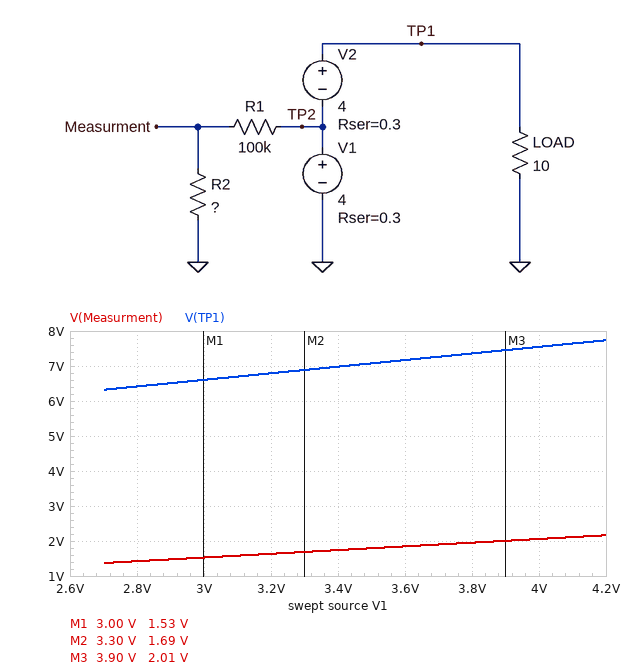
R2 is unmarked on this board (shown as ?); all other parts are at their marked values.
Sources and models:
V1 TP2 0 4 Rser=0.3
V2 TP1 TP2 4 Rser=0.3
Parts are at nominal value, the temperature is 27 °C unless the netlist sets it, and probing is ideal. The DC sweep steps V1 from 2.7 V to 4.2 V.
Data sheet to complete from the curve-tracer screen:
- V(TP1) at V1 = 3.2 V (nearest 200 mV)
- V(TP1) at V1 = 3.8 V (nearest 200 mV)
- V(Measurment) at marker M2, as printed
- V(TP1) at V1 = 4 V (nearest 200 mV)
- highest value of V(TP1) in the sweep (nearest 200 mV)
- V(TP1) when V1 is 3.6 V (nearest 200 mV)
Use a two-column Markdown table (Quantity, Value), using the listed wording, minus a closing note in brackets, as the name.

| Quantity | Value |
|---|---|
| V(TP1) at V1 = 3.2 V | 6.8 V |
| V(TP1) at V1 = 3.8 V | 7.4 V |
| V(Measurment) at marker M2, as printed | 1.69 V |
| V(TP1) at V1 = 4 V | 7.6 V |
| highest value of V(TP1) in the sweep | 7.8 V |
| V(TP1) when V1 is 3.6 V | 7.2 V |
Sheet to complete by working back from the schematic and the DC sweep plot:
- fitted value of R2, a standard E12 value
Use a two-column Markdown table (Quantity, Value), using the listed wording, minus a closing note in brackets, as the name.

| Quantity | Value |
|---|---|
| fitted value of R2, a standard E12 value | 120 kΩ |
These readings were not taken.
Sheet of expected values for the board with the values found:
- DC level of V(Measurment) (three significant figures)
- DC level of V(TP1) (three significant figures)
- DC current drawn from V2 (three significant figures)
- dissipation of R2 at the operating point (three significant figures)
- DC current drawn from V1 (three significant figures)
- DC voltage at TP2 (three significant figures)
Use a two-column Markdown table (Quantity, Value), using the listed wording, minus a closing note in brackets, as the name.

| Quantity | Value |
|---|---|
| DC level of V(Measurment) | 2.06 V |
| DC level of V(TP1) | 7.55 V |
| DC current drawn from V2 | 755 mA |
| dissipation of R2 at the operating point | 35.3 µW |
| DC current drawn from V1 | 755 mA |
| DC voltage at TP2 | 3.77 V |
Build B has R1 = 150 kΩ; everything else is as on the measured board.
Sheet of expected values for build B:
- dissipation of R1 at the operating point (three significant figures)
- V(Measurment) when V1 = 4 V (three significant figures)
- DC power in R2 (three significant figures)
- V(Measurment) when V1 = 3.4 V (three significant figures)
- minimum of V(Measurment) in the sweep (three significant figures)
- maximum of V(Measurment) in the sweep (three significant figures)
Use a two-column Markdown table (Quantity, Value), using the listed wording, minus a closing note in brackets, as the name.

| Quantity | Value |
|---|---|
| dissipation of R1 at the operating point | 29.3 µW |
| V(Measurment) when V1 = 4 V | 1.68 V |
| DC power in R2 | 23.4 µW |
| V(Measurment) when V1 = 3.4 V | 1.42 V |
| minimum of V(Measurment) in the sweep | 1.12 V |
| maximum of V(Measurment) in the sweep | 1.76 V |
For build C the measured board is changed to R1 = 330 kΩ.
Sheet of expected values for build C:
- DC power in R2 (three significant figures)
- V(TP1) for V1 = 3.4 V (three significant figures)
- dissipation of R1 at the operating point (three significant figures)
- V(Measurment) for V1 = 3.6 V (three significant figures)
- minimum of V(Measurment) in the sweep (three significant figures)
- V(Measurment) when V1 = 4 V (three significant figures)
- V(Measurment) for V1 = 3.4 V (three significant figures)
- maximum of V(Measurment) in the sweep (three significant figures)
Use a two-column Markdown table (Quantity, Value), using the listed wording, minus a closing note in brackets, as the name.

| Quantity | Value |
|---|---|
| DC power in R2 | 8.44 µW |
| V(TP1) for V1 = 3.4 V | 6.98 V |
| dissipation of R1 at the operating point | 23.2 µW |
| V(Measurment) for V1 = 3.6 V | 903 mV |
| minimum of V(Measurment) in the sweep | 669 mV |
| V(Measurment) when V1 = 4 V | 1.01 V |
| V(Measurment) for V1 = 3.4 V | 851 mV |
| maximum of V(Measurment) in the sweep | 1.06 V |
